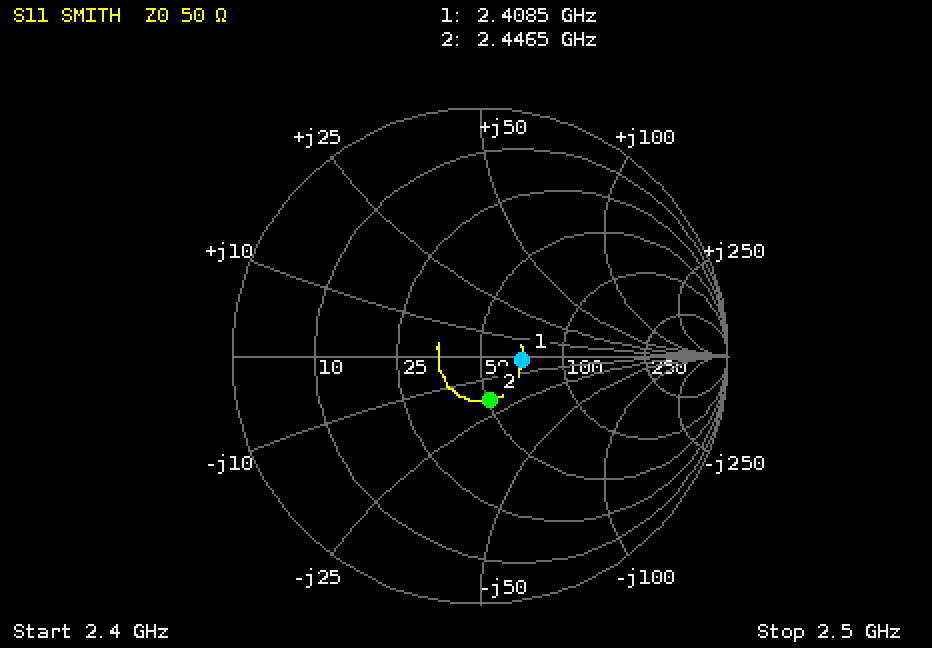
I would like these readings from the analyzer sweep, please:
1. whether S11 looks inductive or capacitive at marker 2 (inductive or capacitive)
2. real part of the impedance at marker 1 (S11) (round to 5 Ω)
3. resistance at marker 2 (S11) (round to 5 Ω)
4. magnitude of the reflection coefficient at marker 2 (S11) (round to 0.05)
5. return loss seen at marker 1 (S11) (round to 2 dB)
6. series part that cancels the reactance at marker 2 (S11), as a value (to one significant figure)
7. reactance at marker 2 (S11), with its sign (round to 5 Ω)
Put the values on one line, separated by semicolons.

capacitive; 70 Ω; 50 Ω; 0.20; 16 dB; 1 nH; -20 Ω
